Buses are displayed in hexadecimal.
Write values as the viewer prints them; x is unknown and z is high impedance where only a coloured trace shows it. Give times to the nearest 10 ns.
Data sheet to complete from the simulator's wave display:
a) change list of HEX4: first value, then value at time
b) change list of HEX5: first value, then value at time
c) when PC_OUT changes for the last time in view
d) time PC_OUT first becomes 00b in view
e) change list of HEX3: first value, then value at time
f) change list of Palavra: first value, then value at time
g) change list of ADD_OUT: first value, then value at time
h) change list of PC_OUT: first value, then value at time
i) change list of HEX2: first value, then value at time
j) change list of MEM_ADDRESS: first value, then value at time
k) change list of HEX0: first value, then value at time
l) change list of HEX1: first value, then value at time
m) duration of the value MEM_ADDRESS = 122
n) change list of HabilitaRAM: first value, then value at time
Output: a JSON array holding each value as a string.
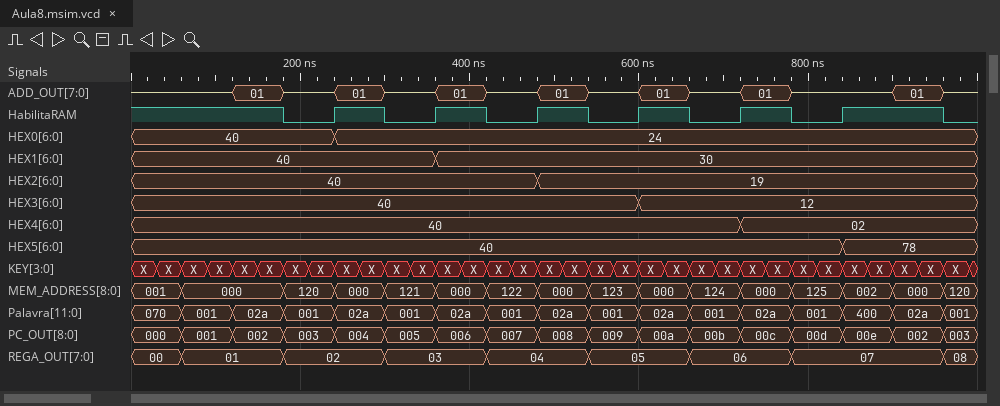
["40, 02 at 720 ns", "40, 78 at 840 ns", "960 ns", "660 ns", "40, 12 at 600 ns", "070, 001 at 60 ns, 02a at 120 ns, 001 at 180 ns, 02a at 240 ns, 001 at 300 ns, 02a at 360 ns, 001 at 420 ns, 02a at 480 ns, 001 at 540 ns, 02a at 600 ns, 001 at 660 ns, 02a at 720 ns, 001 at 780 ns, 400 at 840 ns, 02a at 900 ns, 001 at 960 ns", "z, 01 at 120 ns, z at 180 ns, 01 at 240 ns, z at 300 ns, 01 at 360 ns, z at 420 ns, 01 at 480 ns, z at 540 ns, 01 at 600 ns, z at 660 ns, 01 at 720 ns, z at 780 ns, 01 at 900 ns, z at 960 ns", "000, 001 at 60 ns, 002 at 120 ns, 003 at 180 ns, 004 at 240 ns, 005 at 300 ns, 006 at 360 ns, 007 at 420 ns, 008 at 480 ns, 009 at 540 ns, 00a at 600 ns, 00b at 660 ns, 00c at 720 ns, 00d at 780 ns, 00e at 840 ns, 002 at 900 ns, 003 at 960 ns", "40, 19 at 480 ns", "001, 000 at 60 ns, 120 at 180 ns, 000 at 240 ns, 121 at 300 ns, 000 at 360 ns, 122 at 420 ns, 000 at 480 ns, 123 at 540 ns, 000 at 600 ns, 124 at 660 ns, 000 at 720 ns, 125 at 780 ns, 002 at 840 ns, 000 at 900 ns, 120 at 960 ns", "40, 24 at 240 ns", "40, 30 at 360 ns", "60 ns", "1, 0 at 180 ns, 1 at 240 ns, 0 at 300 ns, 1 at 360 ns, 0 at 420 ns, 1 at 480 ns, 0 at 540 ns, 1 at 600 ns, 0 at 660 ns, 1 at 720 ns, 0 at 780 ns, 1 at 840 ns, 0 at 960 ns"]
